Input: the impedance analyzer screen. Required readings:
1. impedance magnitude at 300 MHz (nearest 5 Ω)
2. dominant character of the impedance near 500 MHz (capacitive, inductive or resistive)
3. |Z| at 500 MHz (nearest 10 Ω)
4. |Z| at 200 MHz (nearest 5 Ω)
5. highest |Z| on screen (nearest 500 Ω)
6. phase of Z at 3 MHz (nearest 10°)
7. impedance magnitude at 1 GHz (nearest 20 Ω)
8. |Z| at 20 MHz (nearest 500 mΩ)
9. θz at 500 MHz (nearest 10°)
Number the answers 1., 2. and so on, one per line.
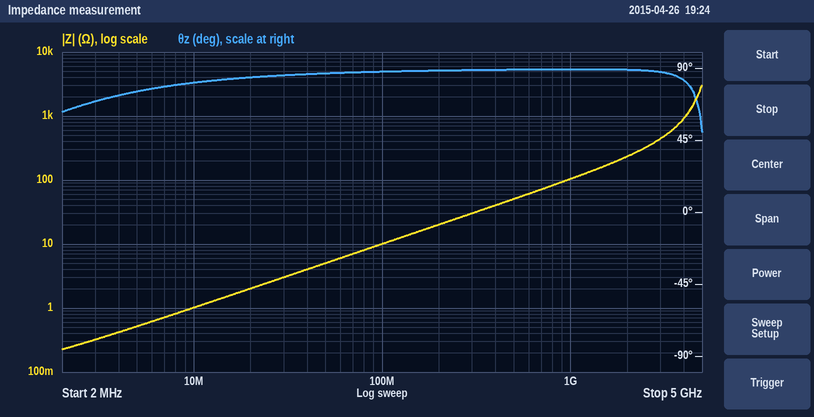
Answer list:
1. 30 Ω
2. inductive
3. 50 Ω
4. 20 Ω
5. 3.0 kΩ
6. 70°
7. 100 Ω
8. 2.0 Ω
9. 90°
